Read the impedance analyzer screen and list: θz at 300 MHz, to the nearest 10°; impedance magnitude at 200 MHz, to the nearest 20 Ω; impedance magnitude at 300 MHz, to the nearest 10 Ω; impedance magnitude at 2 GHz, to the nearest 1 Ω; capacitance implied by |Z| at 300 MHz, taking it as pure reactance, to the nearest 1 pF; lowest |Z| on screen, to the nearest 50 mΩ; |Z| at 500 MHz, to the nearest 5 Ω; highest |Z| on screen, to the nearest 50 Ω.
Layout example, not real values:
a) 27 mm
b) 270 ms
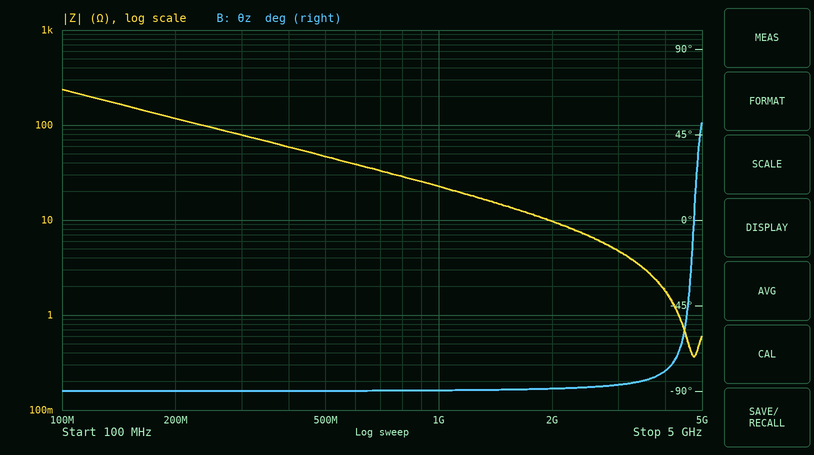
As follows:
a) -90°
b) 120 Ω
c) 80 Ω
d) 10 Ω
e) 7 pF
f) 350 mΩ
g) 45 Ω
h) 250 Ω
